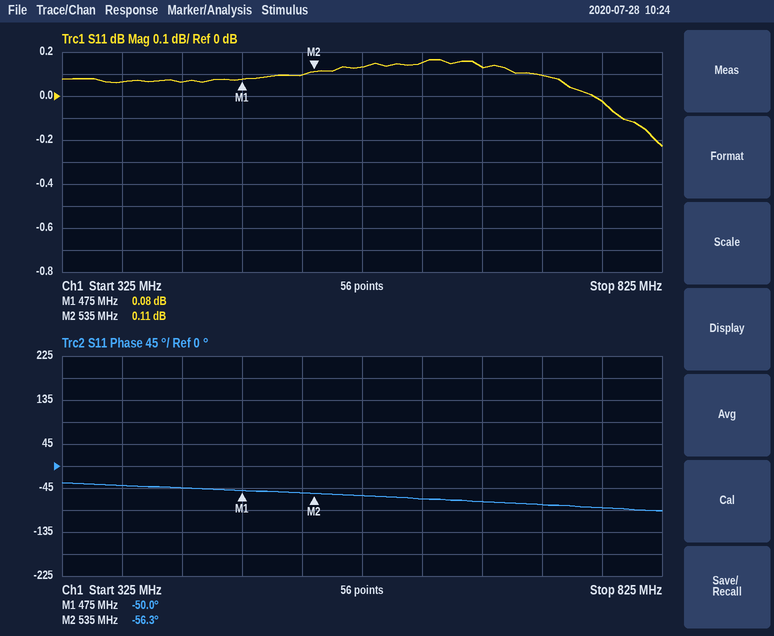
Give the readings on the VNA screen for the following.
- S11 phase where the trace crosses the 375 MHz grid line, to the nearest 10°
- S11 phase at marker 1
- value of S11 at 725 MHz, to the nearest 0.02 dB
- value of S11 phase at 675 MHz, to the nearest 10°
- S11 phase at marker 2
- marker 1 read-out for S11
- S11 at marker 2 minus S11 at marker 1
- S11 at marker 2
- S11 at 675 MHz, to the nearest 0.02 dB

-40°
-50.0°
0.10 dB
-70°
-56.3°
0.08 dB
0.03 dB
0.11 dB
0.14 dB
